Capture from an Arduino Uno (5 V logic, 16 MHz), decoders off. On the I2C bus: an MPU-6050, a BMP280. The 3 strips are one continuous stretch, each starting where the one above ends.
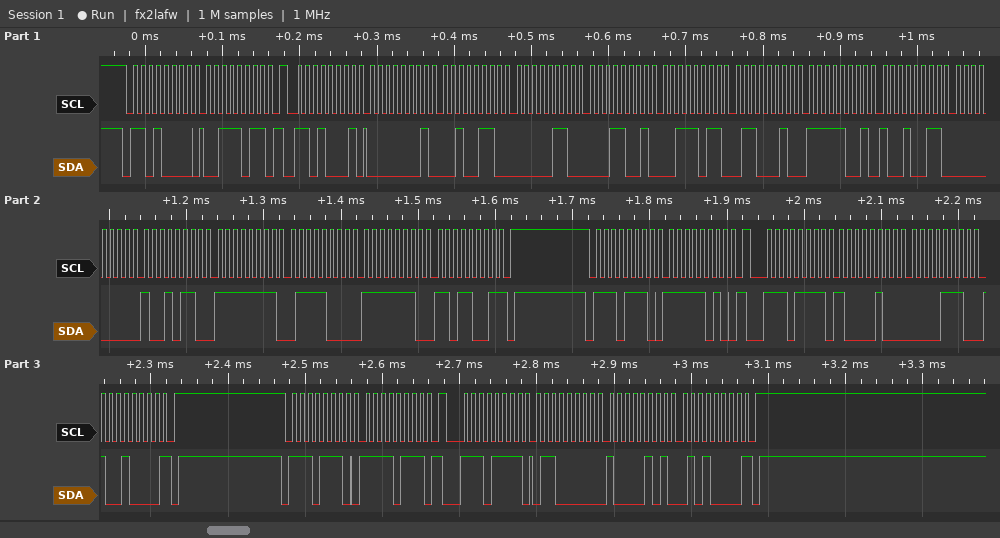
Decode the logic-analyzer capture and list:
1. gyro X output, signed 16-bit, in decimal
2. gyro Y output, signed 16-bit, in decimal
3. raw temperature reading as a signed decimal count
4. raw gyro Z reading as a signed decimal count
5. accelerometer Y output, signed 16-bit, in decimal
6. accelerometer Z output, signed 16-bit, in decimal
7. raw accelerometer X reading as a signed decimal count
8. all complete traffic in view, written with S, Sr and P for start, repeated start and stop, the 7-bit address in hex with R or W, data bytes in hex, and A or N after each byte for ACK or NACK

150
-136
-1645
-295
1561
15202
294
S 68W A 3B A Sr 68R A 01 A 26 A 06 A 19 A 3B A 62 A F9 A 93 A 00 A 96 A FF A 78 A FE A D9 N P S 77W A FA A Sr 77R A 84 A 0E A 90 N P S 77W A F7 A Sr 77R A 60 A 85 A 50 N P
